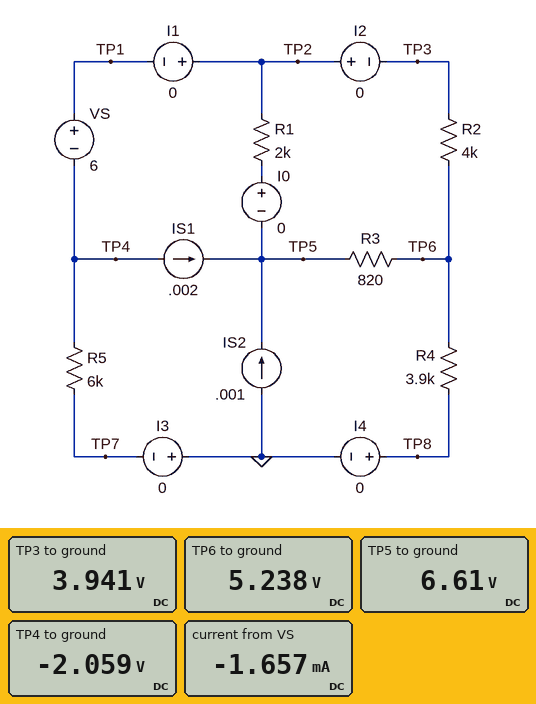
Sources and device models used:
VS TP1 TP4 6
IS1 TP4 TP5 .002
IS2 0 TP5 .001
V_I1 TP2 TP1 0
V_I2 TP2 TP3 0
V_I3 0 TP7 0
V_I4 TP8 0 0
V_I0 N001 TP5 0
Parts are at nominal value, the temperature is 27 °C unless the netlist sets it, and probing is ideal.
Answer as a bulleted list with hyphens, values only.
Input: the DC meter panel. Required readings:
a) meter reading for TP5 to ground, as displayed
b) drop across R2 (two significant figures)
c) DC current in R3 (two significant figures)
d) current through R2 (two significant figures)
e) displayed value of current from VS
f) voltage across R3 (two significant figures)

- 6.61 V
- 1.3 V
- 1.7 mA
- 320 µA
- -1.657 mA
- 1.4 V
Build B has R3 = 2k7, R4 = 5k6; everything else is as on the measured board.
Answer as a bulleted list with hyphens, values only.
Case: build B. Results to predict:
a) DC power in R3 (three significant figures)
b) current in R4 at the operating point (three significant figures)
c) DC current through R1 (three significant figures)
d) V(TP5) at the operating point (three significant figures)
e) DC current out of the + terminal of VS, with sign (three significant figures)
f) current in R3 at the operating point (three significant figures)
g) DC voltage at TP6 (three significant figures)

- 3.78 mW
- 1.07 mA
- 1.82 mA
- 9.20 V
- -1.93 mA
- 1.18 mA
- 6.01 V
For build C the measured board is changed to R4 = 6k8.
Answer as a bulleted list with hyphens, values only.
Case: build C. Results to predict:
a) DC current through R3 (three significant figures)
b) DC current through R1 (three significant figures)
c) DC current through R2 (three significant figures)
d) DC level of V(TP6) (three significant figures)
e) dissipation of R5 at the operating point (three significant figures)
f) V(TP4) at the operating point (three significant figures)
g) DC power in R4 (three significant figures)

- 1.51 mA
- 1.49 mA
- 436 µA
- 7.30 V
- 32.6 µW
- -442 mV
- 7.84 mW
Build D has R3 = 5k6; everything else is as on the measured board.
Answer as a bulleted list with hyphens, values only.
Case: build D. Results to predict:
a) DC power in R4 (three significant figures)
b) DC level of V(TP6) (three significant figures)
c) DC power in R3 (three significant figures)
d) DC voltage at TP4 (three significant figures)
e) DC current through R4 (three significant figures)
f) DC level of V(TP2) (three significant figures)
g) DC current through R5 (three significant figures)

- 4.92 mW
- 4.38 V
- 4.58 mW
- -742 mV
- 1.12 mA
- 5.26 V
- 124 µA
